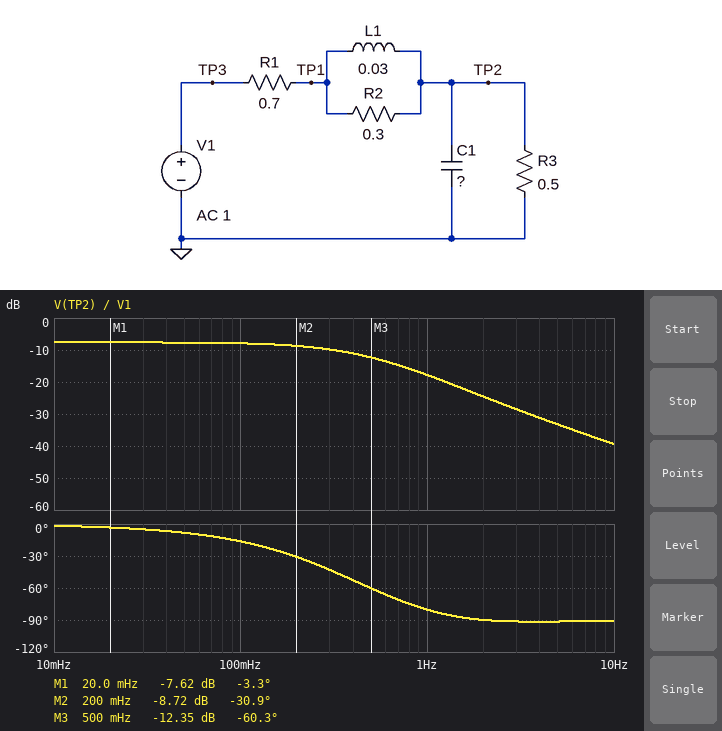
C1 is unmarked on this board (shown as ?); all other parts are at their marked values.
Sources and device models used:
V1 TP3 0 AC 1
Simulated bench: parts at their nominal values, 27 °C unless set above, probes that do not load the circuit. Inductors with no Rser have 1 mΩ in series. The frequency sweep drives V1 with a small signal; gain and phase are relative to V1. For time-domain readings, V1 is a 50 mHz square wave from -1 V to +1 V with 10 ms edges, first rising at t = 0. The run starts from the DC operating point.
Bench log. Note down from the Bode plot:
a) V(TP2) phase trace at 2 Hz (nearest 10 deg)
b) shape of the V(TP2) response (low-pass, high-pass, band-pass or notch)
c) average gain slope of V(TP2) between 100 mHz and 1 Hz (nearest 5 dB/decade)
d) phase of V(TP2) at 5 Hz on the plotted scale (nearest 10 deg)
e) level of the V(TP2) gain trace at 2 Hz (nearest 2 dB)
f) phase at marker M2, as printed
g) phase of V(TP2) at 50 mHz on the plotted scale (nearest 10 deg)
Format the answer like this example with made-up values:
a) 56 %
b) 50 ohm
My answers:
a) -90 deg
b) low-pass
c) -10 dB/decade
d) -90 deg
e) -24 dB
f) -30.9 deg
g) -10 deg
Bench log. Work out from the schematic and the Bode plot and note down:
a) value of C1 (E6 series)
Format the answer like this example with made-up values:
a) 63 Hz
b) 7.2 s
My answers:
a) 1.5 F
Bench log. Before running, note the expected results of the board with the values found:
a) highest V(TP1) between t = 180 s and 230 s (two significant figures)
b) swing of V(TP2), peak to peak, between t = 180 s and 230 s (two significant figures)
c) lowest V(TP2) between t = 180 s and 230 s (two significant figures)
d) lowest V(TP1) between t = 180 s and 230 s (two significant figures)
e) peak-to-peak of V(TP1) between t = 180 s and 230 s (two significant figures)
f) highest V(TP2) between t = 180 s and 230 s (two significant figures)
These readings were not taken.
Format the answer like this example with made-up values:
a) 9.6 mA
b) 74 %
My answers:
a) 420 mV
b) 830 mV
c) -420 mV
d) -420 mV
e) 830 mV
f) 420 mV
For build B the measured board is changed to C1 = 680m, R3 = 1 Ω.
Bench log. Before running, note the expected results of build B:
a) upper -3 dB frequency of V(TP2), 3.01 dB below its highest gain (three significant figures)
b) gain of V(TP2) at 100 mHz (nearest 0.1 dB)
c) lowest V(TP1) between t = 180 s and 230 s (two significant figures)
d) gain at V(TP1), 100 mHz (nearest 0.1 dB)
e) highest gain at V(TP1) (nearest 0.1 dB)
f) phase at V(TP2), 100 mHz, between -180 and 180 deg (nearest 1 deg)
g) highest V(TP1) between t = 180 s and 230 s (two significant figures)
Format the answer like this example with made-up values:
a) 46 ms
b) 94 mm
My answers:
a) 568 mHz
b) -4.7 dB
c) -590 mV
d) -4.8 dB
e) -4.6 dB
f) -11 deg
g) 590 mV
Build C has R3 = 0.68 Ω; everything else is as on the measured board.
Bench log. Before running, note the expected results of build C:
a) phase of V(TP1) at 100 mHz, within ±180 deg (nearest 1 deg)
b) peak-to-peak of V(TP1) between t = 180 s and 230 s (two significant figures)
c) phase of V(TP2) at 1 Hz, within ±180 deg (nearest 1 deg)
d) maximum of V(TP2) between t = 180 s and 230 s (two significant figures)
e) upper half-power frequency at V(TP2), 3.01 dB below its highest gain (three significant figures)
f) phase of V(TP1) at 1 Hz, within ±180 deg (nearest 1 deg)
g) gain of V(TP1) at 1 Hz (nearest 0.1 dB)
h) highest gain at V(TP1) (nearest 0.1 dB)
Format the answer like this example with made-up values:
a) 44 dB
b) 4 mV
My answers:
a) -17 deg
b) 990 mV
c) -83 deg
d) 490 mV
e) 311 mHz
f) 15 deg
g) -17.6 dB
h) -6.1 dB
